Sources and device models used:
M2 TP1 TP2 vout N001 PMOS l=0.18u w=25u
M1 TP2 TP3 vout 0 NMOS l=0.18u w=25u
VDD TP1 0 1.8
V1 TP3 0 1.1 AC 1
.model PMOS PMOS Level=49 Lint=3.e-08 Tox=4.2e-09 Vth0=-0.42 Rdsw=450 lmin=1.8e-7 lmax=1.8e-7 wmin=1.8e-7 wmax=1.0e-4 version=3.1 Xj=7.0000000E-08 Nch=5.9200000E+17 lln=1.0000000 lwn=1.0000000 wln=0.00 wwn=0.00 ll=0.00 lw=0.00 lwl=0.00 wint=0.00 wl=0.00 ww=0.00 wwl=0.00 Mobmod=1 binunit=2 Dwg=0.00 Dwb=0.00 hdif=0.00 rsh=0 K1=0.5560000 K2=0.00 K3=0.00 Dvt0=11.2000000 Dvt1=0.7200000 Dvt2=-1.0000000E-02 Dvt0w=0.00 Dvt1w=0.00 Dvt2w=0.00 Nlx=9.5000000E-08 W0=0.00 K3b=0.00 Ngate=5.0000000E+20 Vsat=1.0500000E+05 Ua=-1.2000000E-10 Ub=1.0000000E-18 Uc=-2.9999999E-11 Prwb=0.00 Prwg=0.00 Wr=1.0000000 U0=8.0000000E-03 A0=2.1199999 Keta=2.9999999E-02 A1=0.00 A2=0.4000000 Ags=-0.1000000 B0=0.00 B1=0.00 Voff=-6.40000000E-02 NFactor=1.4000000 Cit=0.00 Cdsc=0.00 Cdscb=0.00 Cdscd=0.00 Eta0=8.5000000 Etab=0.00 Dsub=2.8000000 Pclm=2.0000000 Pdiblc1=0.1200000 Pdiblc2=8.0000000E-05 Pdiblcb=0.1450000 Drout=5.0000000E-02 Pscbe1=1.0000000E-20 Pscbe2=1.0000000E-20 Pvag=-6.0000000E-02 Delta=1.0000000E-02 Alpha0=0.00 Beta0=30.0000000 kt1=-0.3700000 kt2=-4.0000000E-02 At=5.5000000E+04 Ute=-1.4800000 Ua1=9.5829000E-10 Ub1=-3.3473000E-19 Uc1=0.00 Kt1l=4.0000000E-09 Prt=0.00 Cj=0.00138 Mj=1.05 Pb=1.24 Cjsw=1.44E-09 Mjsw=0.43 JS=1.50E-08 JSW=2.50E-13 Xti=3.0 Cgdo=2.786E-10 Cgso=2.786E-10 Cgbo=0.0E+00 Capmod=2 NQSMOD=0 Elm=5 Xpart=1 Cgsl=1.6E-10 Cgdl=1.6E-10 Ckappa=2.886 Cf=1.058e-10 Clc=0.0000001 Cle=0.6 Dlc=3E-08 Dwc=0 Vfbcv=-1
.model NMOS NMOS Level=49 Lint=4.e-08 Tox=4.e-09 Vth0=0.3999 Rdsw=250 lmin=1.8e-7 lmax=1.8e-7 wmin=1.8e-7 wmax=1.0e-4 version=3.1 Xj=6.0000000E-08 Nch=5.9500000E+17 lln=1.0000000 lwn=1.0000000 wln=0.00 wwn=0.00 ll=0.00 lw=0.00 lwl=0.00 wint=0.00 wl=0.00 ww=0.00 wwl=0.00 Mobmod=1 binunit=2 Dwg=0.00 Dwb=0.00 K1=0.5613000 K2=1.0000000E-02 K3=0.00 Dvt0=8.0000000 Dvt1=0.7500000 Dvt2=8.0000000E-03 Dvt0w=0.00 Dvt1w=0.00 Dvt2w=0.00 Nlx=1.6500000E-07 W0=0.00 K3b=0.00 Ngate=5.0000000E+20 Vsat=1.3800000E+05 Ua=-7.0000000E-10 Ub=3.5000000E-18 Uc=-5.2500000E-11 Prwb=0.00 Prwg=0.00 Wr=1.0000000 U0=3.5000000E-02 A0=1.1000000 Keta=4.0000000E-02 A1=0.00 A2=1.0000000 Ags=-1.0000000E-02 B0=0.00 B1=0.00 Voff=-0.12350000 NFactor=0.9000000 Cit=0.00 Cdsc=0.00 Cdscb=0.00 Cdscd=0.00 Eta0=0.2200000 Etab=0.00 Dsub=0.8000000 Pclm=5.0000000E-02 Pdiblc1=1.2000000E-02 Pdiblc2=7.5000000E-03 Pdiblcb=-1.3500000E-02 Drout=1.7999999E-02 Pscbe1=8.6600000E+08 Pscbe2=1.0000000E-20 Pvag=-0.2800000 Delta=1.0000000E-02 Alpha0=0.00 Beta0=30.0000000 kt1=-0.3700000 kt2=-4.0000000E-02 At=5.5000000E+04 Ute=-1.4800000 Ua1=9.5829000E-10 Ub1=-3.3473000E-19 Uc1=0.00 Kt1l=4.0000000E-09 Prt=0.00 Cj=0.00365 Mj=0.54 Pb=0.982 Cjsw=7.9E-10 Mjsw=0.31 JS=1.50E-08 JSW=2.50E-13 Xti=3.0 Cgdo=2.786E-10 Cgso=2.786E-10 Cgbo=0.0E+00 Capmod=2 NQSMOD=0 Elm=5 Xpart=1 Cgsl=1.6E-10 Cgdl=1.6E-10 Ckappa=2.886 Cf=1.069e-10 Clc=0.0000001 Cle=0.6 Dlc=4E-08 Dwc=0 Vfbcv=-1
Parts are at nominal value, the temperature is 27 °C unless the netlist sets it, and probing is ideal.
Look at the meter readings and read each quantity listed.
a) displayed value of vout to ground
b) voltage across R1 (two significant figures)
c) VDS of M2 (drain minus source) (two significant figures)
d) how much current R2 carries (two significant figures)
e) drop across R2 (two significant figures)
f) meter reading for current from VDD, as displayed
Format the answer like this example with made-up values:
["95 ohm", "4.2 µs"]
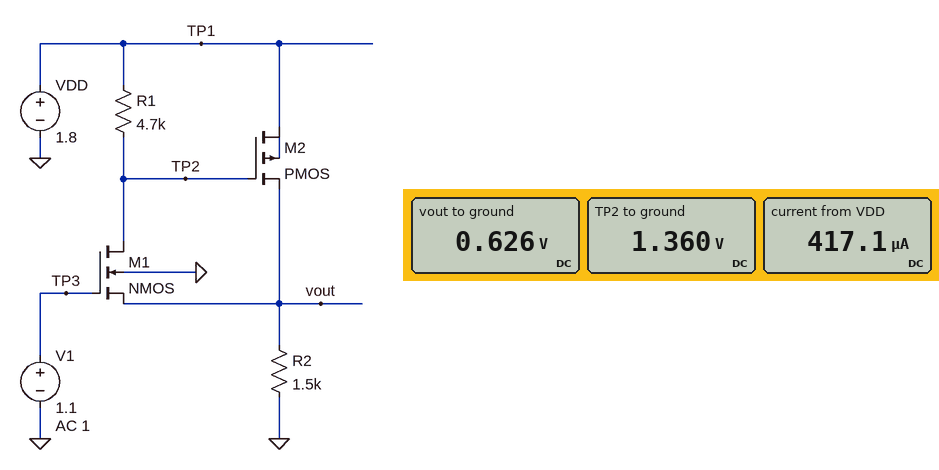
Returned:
["0.626 V", "440 mV", "1.2 V", "420 µA", "630 mV", "417.1 µA"]
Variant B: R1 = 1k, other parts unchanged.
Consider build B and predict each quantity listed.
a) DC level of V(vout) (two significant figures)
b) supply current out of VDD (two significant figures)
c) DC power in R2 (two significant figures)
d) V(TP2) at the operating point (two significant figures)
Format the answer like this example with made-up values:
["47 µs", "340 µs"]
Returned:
["570 mV", "380 µA", "220 µW", "1.5 V"]
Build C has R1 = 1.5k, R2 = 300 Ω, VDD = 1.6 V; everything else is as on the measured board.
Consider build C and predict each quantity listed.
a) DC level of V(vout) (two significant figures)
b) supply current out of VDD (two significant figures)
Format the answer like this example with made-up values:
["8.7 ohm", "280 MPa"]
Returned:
["510 mV", "1.7 mA"]
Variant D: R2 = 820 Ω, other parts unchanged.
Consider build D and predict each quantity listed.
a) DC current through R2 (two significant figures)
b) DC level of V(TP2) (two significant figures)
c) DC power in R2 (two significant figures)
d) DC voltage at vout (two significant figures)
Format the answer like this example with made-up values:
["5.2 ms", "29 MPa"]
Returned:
["750 µA", "1.3 V", "460 µW", "610 mV"]
